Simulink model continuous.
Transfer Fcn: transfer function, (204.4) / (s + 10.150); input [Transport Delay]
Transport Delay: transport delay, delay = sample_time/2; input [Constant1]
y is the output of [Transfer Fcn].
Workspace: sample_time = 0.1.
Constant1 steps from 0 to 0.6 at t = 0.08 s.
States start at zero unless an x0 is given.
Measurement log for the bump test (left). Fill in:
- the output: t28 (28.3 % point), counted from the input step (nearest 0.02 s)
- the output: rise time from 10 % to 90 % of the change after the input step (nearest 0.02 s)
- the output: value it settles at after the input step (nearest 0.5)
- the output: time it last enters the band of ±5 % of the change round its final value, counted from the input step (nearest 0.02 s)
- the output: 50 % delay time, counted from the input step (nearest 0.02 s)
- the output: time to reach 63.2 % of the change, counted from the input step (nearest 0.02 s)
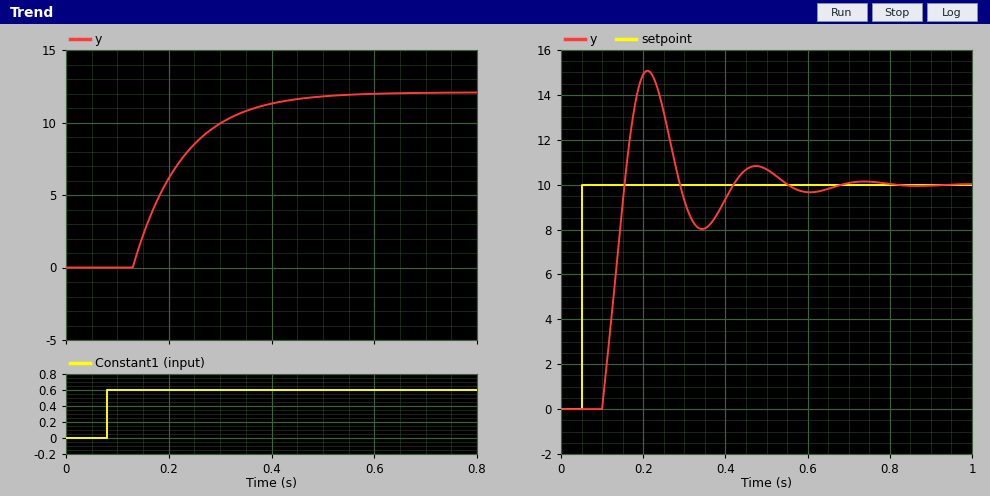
0.08 s
0.22 s
12.0
0.34 s
0.12 s
0.14 s
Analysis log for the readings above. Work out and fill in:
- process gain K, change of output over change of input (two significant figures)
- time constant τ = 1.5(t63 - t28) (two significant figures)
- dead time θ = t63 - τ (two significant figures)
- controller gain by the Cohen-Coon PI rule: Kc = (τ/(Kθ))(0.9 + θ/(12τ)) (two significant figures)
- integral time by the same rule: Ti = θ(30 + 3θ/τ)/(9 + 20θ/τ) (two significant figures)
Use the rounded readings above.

20
0.090 s
0.050 s
0.085
0.079 s
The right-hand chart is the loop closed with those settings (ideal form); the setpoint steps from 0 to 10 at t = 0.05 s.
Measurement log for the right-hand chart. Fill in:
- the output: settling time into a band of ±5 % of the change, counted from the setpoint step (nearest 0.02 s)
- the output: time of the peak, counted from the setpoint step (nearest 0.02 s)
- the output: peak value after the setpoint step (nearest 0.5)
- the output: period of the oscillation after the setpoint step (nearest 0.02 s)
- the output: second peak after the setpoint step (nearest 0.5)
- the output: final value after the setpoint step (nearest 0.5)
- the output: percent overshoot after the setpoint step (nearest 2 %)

0.46 s
0.16 s
15.0
0.26 s
11.0
10.0
50 %
